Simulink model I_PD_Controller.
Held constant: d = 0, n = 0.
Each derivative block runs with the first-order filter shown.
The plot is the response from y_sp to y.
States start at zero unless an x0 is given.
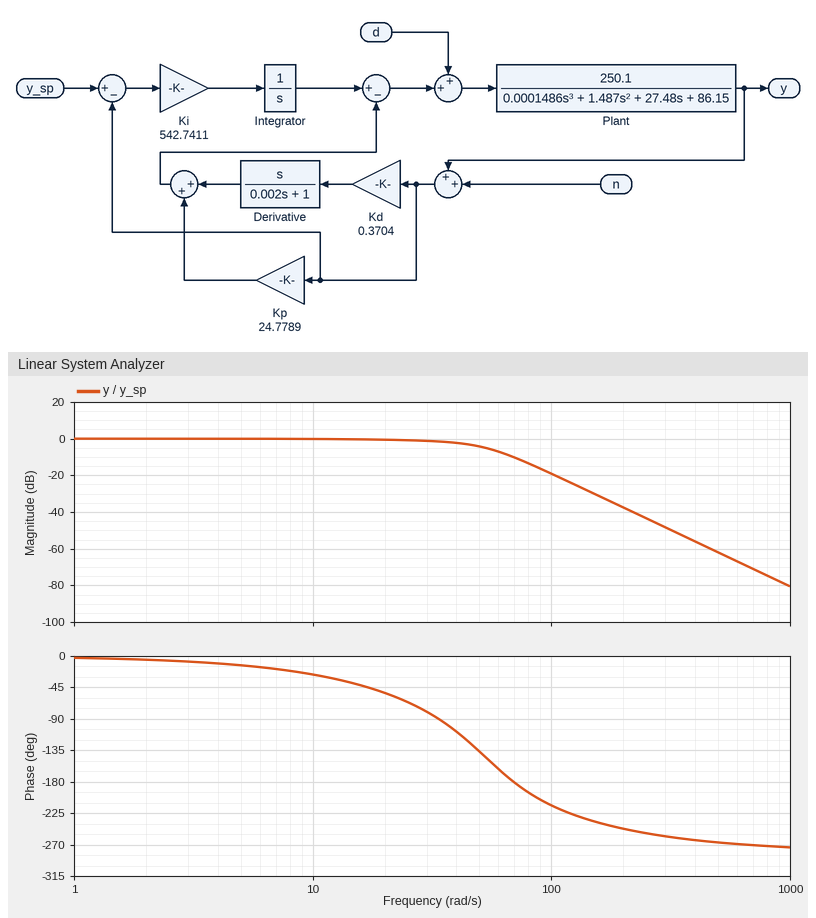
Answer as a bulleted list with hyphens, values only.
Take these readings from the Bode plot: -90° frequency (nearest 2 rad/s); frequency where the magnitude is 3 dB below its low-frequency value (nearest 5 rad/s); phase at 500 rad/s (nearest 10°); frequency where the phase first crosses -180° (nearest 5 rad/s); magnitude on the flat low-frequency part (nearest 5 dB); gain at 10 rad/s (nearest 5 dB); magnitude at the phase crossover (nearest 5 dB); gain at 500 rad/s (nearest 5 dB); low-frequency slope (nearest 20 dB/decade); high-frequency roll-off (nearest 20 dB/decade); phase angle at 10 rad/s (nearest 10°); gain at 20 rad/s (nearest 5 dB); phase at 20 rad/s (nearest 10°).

- 34 rad/s
- 45 rad/s
- -270°
- 70 rad/s
- 0 dB
- 0 dB
- -10 dB
- -60 dB
- 0 dB/decade
- -60 dB/decade
- -30°
- 0 dB
- -50°
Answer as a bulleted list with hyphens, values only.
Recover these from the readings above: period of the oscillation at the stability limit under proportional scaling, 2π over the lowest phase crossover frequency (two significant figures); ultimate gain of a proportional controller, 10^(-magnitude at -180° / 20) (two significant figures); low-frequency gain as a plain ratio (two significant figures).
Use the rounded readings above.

- 0.090 s
- 3.2
- 1.0
